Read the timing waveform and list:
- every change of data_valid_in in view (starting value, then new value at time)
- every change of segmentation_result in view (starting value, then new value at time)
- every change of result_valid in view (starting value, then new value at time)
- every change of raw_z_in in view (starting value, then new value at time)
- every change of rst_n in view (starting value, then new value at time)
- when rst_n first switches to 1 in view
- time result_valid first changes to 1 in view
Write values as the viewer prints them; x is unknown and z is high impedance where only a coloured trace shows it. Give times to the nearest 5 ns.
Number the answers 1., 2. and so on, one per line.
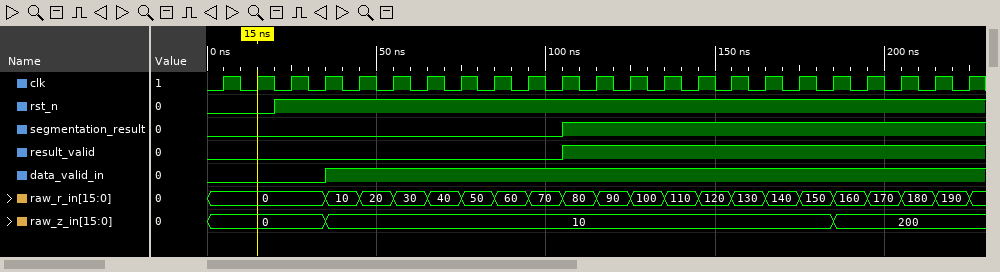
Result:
1. 0, 1 at 35 ns
2. 0, 1 at 105 ns
3. 0, 1 at 105 ns
4. 0, 10 at 35 ns, 200 at 185 ns
5. 0, 1 at 20 ns
6. 20 ns
7. 105 ns
